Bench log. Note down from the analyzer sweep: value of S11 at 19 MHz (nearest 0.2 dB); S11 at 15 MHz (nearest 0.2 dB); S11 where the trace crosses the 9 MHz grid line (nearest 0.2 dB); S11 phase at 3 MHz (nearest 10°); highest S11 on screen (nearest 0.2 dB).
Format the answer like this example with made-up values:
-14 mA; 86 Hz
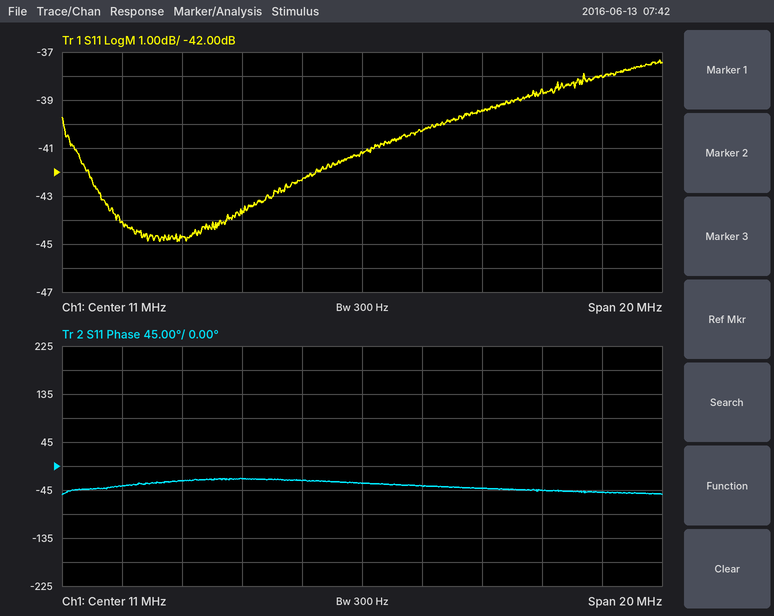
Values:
-38.0 dB; -39.4 dB; -42.4 dB; -40°; -37.4 dB
